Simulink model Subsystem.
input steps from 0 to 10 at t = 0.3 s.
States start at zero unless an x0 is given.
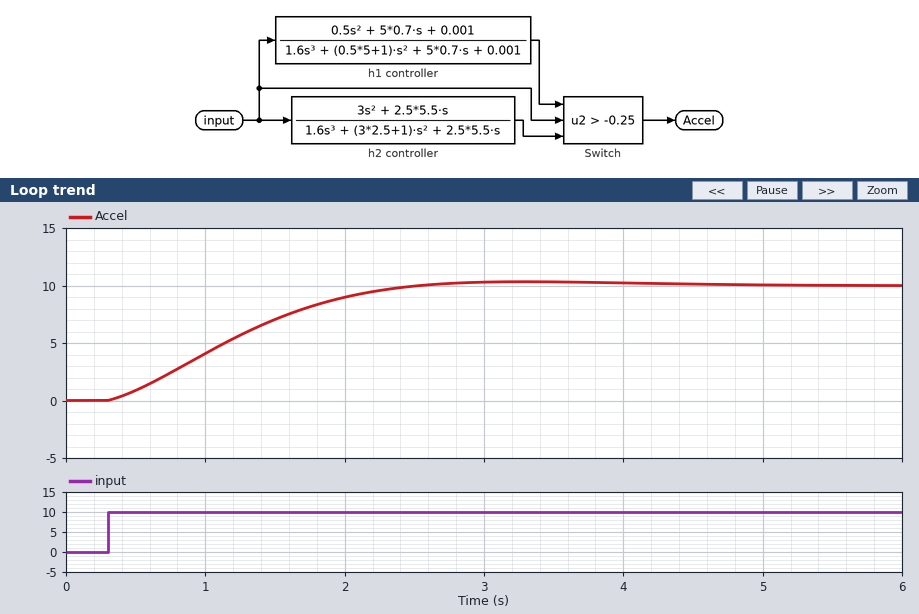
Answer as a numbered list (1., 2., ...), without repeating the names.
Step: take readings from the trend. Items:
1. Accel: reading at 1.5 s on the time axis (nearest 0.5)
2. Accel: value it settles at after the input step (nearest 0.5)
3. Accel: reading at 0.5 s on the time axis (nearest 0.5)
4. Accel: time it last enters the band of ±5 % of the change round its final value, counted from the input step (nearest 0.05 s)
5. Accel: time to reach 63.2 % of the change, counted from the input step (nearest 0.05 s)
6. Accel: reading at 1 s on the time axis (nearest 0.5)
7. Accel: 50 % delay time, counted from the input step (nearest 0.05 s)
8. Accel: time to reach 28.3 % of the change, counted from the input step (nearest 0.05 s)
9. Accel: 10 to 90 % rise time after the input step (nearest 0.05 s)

1. 7.0
2. 10.0
3. 1.0
4. 1.90 s
5. 1.05 s
6. 4.0
7. 0.85 s
8. 0.50 s
9. 1.50 s
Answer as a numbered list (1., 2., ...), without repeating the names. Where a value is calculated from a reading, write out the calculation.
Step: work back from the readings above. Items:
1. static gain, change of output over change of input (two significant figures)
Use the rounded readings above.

1. (10 - 0) / (10 - 0) = 1.0
